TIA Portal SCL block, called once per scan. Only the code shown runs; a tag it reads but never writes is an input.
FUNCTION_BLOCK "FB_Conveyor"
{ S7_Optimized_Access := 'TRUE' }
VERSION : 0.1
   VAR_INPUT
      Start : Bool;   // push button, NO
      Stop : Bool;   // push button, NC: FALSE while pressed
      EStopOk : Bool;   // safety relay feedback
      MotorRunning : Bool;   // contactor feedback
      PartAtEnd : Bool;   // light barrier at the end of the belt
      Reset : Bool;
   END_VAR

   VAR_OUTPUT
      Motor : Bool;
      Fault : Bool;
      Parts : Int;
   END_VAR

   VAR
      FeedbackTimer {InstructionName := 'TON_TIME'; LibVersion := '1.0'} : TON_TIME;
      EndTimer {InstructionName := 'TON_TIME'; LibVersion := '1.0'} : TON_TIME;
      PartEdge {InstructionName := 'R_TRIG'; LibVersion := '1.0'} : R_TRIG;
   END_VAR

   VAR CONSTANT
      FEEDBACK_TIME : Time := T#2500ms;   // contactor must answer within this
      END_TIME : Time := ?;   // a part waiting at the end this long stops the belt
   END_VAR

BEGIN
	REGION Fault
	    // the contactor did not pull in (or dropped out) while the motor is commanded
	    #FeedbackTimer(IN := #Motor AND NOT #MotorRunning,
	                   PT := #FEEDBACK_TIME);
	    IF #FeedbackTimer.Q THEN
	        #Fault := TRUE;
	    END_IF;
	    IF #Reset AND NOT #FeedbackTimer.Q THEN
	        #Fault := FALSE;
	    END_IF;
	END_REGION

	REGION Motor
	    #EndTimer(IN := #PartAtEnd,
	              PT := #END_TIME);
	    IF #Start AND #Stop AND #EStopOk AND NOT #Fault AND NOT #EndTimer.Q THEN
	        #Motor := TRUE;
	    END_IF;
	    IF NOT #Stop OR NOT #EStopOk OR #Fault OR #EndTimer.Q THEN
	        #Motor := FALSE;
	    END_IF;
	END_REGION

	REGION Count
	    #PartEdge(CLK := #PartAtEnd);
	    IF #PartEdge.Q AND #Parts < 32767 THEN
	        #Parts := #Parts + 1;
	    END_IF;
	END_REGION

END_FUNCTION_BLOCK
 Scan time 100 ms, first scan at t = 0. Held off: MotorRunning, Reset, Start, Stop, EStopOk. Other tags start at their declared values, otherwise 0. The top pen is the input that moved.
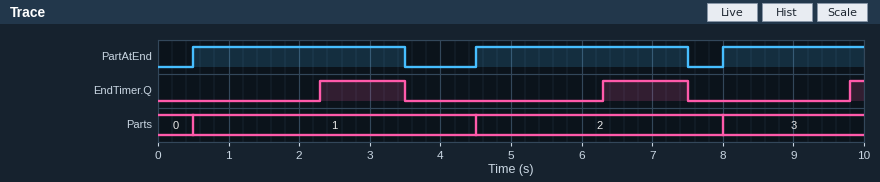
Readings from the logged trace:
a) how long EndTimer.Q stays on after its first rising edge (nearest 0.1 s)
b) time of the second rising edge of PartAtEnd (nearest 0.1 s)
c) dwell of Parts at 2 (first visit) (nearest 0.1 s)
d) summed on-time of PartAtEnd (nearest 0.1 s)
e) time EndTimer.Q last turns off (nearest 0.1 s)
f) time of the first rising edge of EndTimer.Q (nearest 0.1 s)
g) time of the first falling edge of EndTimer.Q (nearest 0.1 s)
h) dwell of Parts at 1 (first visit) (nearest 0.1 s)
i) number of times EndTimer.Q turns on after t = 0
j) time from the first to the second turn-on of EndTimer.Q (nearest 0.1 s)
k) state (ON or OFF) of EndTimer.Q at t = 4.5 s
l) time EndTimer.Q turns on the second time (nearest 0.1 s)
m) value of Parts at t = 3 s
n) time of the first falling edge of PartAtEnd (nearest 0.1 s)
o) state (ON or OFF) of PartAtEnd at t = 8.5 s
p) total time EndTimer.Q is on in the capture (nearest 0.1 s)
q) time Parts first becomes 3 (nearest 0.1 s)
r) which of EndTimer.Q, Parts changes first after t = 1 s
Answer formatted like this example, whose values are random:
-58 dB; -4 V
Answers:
1.2 s; 4.5 s; 3.5 s; 8.0 s; 7.5 s; 2.3 s; 3.5 s; 4.0 s; 3; 4.0 s; OFF; 6.3 s; 1; 3.5 s; ON; 2.6 s; 8.0 s; EndTimer.Q
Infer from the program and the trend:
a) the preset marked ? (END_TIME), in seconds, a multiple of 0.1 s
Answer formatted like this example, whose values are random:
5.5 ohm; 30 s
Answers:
1.8 s
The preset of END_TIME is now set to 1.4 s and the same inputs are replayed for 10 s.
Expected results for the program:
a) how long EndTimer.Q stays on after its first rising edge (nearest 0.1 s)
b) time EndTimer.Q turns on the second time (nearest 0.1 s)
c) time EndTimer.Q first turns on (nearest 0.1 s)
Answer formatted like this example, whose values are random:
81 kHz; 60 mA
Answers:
1.6 s; 5.9 s; 1.9 s
